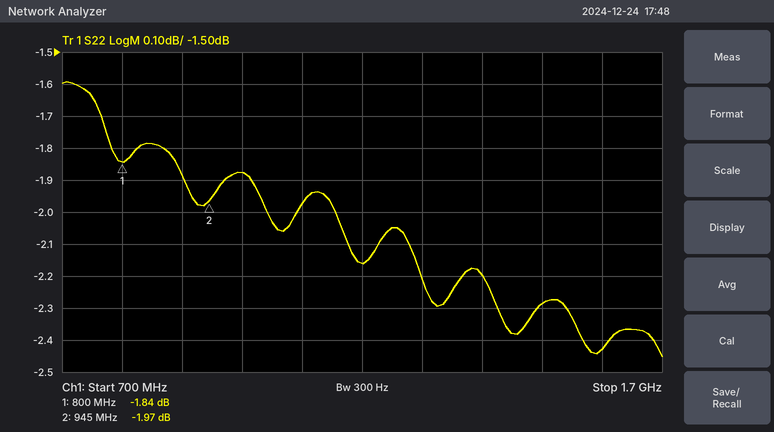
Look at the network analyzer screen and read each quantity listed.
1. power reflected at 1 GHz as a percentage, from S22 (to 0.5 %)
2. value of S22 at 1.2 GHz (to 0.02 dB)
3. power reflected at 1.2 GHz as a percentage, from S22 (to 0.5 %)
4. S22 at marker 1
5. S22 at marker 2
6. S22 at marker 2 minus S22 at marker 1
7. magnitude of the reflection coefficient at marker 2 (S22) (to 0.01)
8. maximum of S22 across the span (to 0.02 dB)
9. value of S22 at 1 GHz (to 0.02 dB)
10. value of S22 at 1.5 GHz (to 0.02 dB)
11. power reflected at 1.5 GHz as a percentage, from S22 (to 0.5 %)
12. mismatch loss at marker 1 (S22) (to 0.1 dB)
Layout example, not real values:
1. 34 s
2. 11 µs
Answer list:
1. 65.0 %
2. -2.16 dB
3. 61.0 %
4. -1.84 dB
5. -1.97 dB
6. -0.13 dB
7. 0.80
8. -1.60 dB
9. -1.88 dB
10. -2.28 dB
11. 59.0 %
12. 4.6 dB
